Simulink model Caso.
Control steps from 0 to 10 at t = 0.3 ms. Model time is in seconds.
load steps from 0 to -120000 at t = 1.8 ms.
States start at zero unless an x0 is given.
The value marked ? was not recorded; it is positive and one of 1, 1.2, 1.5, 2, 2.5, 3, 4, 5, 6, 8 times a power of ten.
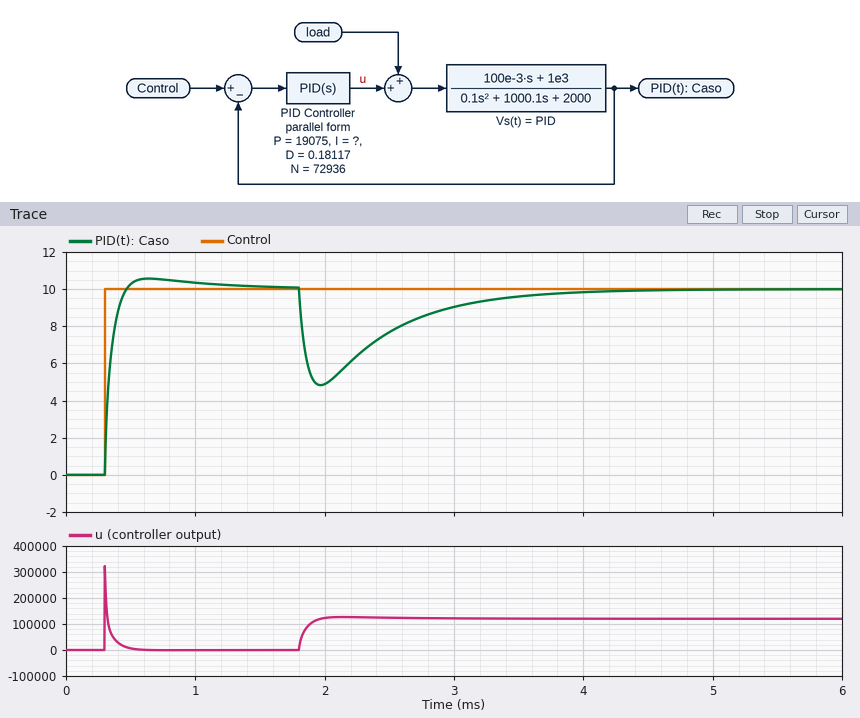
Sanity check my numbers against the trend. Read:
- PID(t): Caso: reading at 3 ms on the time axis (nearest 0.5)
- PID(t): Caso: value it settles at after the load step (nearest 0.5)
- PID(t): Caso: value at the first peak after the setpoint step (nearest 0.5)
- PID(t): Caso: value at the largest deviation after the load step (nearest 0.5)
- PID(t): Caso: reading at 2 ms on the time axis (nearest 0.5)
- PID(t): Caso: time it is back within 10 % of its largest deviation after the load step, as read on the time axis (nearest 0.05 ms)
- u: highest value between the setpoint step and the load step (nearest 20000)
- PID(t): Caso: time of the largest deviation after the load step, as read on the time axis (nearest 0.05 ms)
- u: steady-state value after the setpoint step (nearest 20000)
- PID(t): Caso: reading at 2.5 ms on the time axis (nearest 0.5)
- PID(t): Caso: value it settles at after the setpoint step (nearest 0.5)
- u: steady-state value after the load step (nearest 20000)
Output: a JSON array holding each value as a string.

["9.0", "10.0", "10.5", "5.0", "5.0", "3.35 ms", "320000", "1.95 ms", "0", "7.5", "10.0", "120000"]
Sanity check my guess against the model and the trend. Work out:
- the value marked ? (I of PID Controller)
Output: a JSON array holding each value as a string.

["3e+07"]
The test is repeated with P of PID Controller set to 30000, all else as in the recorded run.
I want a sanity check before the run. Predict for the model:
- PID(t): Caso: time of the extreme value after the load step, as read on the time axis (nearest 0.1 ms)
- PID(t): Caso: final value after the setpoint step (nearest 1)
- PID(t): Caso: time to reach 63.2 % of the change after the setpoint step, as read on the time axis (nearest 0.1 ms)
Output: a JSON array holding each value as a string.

["1.9 ms", "10", "0.3 ms"]
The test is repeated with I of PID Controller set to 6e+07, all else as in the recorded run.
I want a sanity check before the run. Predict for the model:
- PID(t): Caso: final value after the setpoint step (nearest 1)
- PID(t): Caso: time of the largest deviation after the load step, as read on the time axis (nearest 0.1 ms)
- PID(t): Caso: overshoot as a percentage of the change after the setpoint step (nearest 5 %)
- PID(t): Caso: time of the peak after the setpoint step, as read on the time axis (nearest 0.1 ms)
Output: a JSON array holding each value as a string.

["10", "1.9 ms", "10 %", "0.6 ms"]
